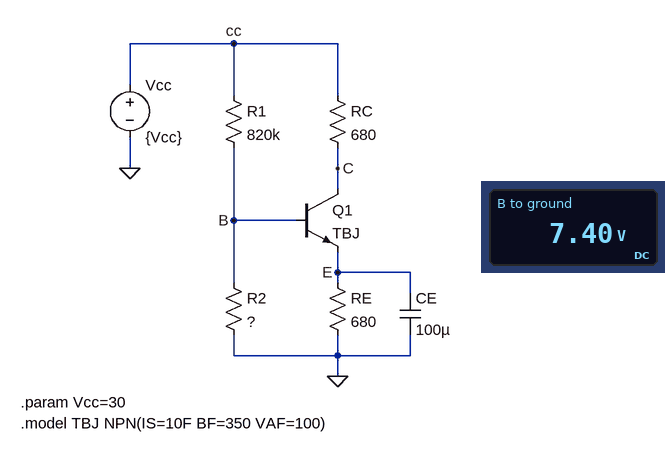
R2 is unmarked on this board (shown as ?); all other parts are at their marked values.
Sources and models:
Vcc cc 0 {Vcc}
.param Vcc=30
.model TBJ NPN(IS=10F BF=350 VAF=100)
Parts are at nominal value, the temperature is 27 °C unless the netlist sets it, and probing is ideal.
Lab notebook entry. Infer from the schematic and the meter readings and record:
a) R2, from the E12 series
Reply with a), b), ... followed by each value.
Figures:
a) 2.2 MΩ
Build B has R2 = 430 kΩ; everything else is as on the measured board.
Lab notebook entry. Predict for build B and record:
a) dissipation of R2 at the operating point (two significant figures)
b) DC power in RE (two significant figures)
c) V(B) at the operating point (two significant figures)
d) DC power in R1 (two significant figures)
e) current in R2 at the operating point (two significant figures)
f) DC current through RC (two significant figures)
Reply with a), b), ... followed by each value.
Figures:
a) 71 µW
b) 34 mW
c) 5.5 V
d) 730 µW
e) 13 µA
f) 7.1 mA
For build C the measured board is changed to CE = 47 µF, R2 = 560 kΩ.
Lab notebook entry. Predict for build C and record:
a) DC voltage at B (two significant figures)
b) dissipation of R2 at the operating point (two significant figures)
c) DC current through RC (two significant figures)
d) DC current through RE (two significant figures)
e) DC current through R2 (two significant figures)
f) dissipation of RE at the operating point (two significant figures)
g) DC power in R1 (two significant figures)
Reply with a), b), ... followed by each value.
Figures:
a) 6.0 V
b) 64 µW
c) 7.7 mA
d) 7.8 mA
e) 11 µA
f) 41 mW
g) 700 µW
